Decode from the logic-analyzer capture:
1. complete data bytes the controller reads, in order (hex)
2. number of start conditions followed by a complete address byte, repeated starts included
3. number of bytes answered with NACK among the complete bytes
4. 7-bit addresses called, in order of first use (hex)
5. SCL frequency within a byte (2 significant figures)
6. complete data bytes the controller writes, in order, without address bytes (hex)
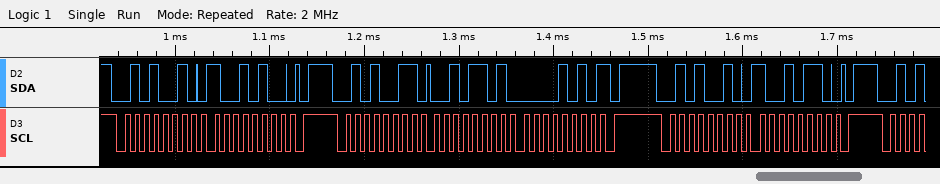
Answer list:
2D 0A
3
1
0x29
100 kHz
94 96
